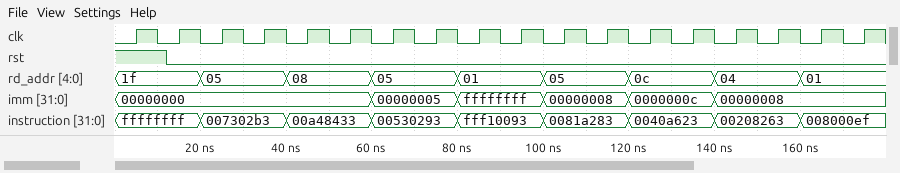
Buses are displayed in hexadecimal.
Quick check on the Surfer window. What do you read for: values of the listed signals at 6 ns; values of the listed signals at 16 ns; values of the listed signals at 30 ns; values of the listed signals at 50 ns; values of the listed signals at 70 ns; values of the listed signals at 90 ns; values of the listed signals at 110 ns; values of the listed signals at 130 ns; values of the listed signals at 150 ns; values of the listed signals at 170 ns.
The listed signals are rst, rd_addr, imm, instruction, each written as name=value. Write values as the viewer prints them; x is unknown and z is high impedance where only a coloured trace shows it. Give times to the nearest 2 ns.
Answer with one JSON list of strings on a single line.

["rst=1, rd_addr=1f, imm=00000000, instruction=ffffffff", "rst=0, rd_addr=1f, imm=00000000, instruction=ffffffff", "rst=0, rd_addr=05, imm=00000000, instruction=007302b3", "rst=0, rd_addr=08, imm=00000000, instruction=00a48433", "rst=0, rd_addr=05, imm=00000005, instruction=00530293", "rst=0, rd_addr=01, imm=ffffffff, instruction=fff10093", "rst=0, rd_addr=05, imm=00000008, instruction=0081a283", "rst=0, rd_addr=0c, imm=0000000c, instruction=0040a623", "rst=0, rd_addr=04, imm=00000008, instruction=00208263", "rst=0, rd_addr=01, imm=00000008, instruction=008000ef"]
